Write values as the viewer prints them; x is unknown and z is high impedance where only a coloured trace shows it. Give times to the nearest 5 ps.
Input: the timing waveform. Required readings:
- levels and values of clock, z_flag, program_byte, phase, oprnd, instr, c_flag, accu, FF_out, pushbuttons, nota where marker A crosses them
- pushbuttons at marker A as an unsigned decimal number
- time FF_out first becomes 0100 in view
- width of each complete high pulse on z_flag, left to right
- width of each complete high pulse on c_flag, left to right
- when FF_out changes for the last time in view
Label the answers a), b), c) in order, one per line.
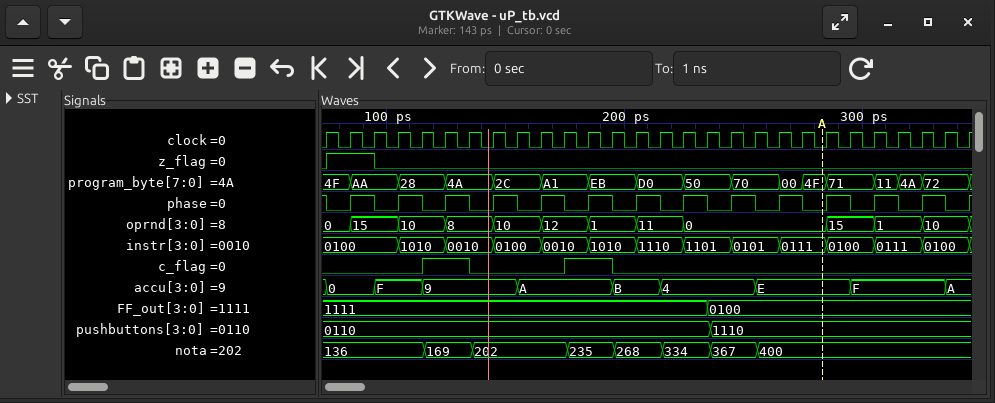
a) clock=0, z_flag=0, program_byte=4F, phase=0, oprnd=0, instr=0111, c_flag=0, accu=E, FF_out=0100, pushbuttons=1110, nota=400
b) 14
c) 235 ps
d) 20 ps
e) 20 ps, 20 ps
f) 235 ps
